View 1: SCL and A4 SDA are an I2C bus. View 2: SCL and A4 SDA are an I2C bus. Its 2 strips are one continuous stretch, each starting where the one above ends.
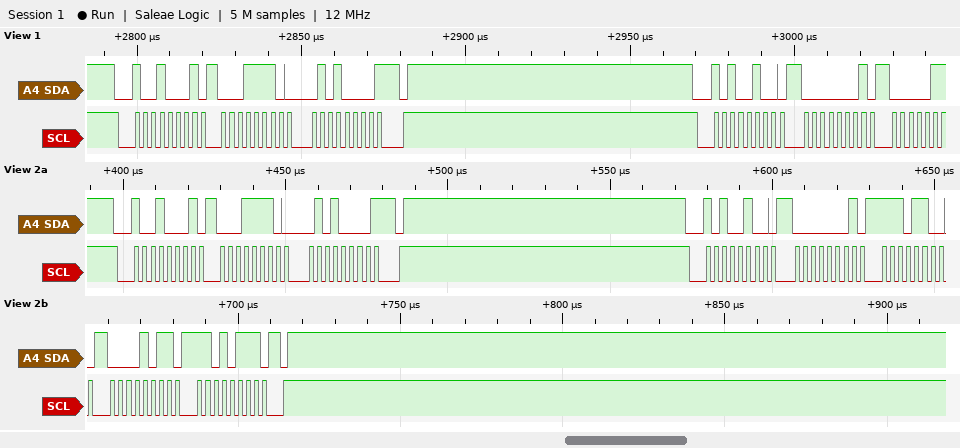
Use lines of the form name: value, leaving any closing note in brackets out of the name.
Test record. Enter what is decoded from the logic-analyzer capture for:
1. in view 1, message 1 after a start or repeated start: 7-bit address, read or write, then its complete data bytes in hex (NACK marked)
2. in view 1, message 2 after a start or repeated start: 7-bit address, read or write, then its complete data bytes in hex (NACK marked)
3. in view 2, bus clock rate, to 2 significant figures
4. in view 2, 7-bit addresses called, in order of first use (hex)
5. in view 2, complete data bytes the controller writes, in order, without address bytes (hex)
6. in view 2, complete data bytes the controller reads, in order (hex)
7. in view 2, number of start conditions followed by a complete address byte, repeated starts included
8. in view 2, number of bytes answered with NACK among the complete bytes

in view 1, message 1 after a start or repeated start: 7-bit address, read or write, then its complete data bytes in hex: 0x48 read: 1E 50 NACK
in view 1, message 2 after a start or repeated start: 7-bit address, read or write, then its complete data bytes in hex: 0x52 write: 01
in view 2, bus clock rate, to 2 significant figures: 400 kHz
in view 2, 7-bit addresses called, in order of first use: 0x48 0x52
in view 2, complete data bytes the controller writes, in order, without address bytes: 01 EC 0B D7
in view 2, complete data bytes the controller reads, in order: 1E 50
in view 2, number of start conditions followed by a complete address byte, repeated starts included: 2
in view 2, number of bytes answered with NACK among the complete bytes: 1
